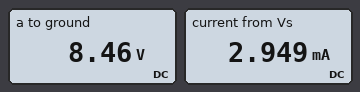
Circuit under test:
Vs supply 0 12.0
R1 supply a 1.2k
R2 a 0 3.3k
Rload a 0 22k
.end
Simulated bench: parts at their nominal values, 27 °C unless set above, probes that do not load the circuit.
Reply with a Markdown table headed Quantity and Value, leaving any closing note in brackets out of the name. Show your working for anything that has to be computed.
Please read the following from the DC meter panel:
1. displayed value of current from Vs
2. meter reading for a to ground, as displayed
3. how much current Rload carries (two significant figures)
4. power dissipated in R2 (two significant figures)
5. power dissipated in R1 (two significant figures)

| Quantity | Value |
|---|---|
| displayed value of current from Vs | 2.949 mA |
| meter reading for a to ground, as displayed | 8.46 V |
| how much current Rload carries | (8.46 V) / 22 kΩ = 380 µA |
| power dissipated in R2 | (8.46 V)^2 / 3.3 kΩ = 22 mW |
| power dissipated in R1 | (12 V - 8.46 V)^2 / 1.2 kΩ = 10 mW |
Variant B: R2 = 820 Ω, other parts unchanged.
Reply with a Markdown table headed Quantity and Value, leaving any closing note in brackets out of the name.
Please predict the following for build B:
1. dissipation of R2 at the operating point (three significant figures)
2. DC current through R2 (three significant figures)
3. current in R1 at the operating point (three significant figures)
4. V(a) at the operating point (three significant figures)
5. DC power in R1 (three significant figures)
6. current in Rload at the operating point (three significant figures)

| Quantity | Value |
|---|---|
| dissipation of R2 at the operating point | 27.7 mW |
| DC current through R2 | 5.81 mA |
| current in R1 at the operating point | 6.03 mA |
| V(a) at the operating point | 4.77 V |
| DC power in R1 | 43.6 mW |
| current in Rload at the operating point | 217 µA |
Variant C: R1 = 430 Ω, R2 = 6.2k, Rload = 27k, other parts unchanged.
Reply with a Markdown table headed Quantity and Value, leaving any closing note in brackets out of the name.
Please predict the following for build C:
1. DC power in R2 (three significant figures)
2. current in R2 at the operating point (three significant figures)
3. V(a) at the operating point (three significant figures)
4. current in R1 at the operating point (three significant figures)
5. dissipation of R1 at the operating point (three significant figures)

| Quantity | Value |
|---|---|
| DC power in R2 | 19.7 mW |
| current in R2 at the operating point | 1.78 mA |
| V(a) at the operating point | 11.1 V |
| current in R1 at the operating point | 2.19 mA |
| dissipation of R1 at the operating point | 2.07 mW |
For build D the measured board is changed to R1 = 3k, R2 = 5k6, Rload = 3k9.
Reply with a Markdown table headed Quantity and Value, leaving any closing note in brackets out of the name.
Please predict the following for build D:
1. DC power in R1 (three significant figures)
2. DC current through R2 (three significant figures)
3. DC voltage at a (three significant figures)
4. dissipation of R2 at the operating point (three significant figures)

| Quantity | Value |
|---|---|
| DC power in R1 | 15.4 mW |
| DC current through R2 | 930 µA |
| DC voltage at a | 5.21 V |
| dissipation of R2 at the operating point | 4.84 mW |
